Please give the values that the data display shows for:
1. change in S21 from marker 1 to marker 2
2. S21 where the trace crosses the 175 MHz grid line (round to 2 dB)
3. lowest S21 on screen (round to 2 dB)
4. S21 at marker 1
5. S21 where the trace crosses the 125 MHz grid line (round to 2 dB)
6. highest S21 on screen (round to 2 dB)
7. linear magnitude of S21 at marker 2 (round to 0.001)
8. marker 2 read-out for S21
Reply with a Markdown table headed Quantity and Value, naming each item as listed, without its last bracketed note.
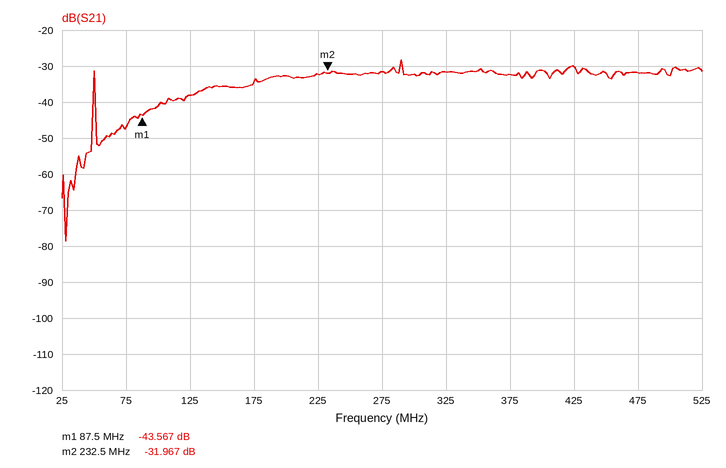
| Quantity | Value |
|---|---|
| change in S21 from marker 1 to marker 2 | 11.600 dB |
| S21 where the trace crosses the 175 MHz grid line | -34 dB |
| lowest S21 on screen | -78 dB |
| S21 at marker 1 | -43.567 dB |
| S21 where the trace crosses the 125 MHz grid line | -38 dB |
| highest S21 on screen | -28 dB |
| linear magnitude of S21 at marker 2 | 0.025 |
| marker 2 read-out for S21 | -31.967 dB |
